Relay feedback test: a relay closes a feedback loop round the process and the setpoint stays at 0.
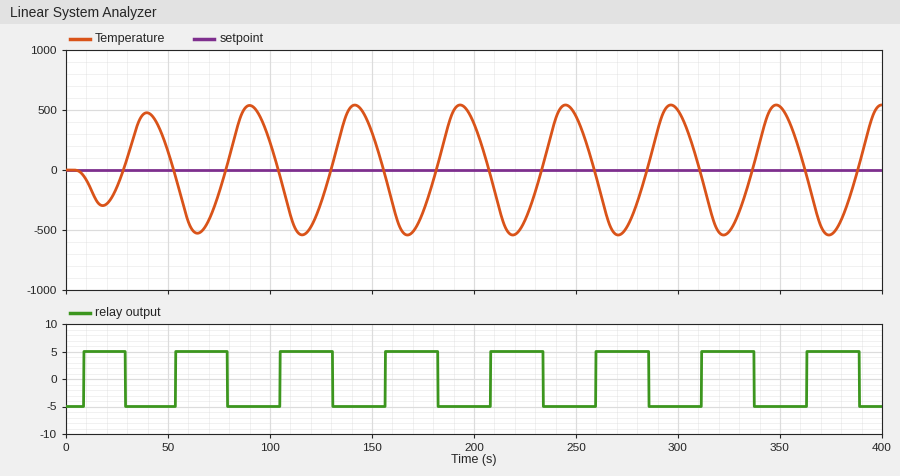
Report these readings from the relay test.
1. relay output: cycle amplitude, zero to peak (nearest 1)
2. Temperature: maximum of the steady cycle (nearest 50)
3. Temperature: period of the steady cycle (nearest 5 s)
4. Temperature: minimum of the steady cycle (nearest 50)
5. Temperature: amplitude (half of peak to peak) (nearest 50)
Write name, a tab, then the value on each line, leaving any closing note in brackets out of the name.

relay output: cycle amplitude, zero to peak	5
Temperature: maximum of the steady cycle	550
Temperature: period of the steady cycle	50 s
Temperature: minimum of the steady cycle	-550
Temperature: amplitude (half of peak to peak)	550
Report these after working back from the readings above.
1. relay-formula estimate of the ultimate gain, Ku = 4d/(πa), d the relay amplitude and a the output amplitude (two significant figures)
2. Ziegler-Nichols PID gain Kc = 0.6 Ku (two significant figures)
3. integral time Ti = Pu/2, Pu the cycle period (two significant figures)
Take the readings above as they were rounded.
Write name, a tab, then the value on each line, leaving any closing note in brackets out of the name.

relay-formula estimate of the ultimate gain, Ku = 4d/(πa), d the relay amplitude and a the output amplitude	0.012
Ziegler-Nichols PID gain Kc = 0.6 Ku	0.0072
integral time Ti = Pu/2, Pu the cycle period	25 s
